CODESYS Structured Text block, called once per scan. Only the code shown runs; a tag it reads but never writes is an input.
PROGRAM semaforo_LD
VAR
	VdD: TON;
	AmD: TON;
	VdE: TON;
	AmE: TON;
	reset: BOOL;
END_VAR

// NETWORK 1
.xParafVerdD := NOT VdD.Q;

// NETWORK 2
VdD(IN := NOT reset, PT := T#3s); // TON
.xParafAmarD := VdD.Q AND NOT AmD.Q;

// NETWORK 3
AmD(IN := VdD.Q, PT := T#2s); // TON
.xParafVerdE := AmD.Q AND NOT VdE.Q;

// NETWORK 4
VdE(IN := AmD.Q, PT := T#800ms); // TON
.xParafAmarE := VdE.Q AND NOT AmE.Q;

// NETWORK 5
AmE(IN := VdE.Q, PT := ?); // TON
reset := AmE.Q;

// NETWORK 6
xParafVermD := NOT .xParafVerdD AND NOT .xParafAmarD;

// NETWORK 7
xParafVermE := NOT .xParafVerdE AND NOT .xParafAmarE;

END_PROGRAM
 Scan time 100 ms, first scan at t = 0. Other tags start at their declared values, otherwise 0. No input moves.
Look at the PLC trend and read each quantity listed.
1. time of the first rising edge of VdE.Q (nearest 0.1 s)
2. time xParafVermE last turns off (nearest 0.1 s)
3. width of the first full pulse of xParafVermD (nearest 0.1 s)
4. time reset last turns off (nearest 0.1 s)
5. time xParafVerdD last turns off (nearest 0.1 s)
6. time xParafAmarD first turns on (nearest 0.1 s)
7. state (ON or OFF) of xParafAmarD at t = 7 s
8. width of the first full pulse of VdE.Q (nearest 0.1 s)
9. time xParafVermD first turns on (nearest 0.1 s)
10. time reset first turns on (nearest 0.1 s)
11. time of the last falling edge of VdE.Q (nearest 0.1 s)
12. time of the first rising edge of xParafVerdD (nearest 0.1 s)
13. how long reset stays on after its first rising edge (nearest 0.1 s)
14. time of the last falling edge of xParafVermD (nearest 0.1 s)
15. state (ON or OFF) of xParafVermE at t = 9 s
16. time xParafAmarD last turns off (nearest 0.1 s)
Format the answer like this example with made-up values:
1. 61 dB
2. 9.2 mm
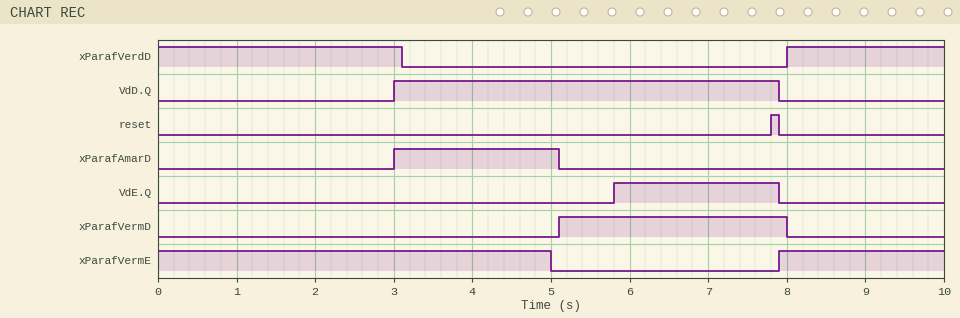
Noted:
1. 5.8 s
2. 5.0 s
3. 2.9 s
4. 7.9 s
5. 3.1 s
6. 3.0 s
7. OFF
8. 2.1 s
9. 5.1 s
10. 7.8 s
11. 7.9 s
12. 8.0 s
13. 0.1 s
14. 8.0 s
15. ON
16. 5.1 s
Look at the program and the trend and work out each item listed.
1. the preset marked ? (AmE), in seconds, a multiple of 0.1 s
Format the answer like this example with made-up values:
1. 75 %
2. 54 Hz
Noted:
1. 2.0 s
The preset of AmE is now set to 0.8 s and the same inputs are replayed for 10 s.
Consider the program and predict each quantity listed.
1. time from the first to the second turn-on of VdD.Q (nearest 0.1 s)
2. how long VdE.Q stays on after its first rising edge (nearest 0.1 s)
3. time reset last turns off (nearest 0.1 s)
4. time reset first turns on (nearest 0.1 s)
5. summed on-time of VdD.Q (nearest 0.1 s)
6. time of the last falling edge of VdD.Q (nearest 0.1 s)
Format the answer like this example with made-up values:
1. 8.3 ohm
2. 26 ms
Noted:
1. 6.8 s
2. 0.9 s
3. 6.7 s
4. 6.6 s
5. 3.9 s
6. 6.7 s
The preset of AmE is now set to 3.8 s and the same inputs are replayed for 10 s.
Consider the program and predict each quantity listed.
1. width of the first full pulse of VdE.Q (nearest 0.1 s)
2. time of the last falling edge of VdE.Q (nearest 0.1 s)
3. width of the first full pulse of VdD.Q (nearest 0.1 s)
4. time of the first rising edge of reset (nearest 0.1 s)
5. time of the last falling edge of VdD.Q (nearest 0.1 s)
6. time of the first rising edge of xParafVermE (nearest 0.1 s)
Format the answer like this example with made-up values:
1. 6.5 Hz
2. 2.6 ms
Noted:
1. 3.9 s
2. 9.7 s
3. 6.7 s
4. 9.6 s
5. 9.7 s
6. 9.7 s
